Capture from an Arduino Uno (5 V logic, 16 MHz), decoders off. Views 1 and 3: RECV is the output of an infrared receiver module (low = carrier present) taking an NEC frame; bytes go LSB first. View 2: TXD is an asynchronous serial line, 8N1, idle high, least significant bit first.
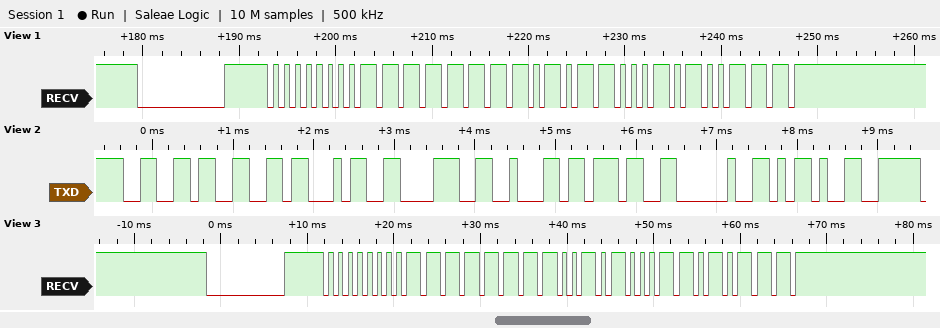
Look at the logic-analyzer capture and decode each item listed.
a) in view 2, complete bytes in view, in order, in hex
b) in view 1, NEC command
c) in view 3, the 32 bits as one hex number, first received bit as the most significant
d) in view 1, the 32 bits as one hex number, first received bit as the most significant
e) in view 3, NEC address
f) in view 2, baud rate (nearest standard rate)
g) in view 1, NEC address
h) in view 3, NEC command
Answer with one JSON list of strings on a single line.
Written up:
["66 66 34 38 62 37 20 2D", "0x1A", "0x00FF28D7", "0x00FF58A7", "0x00", "9600 baud", "0x00", "0x14"]
